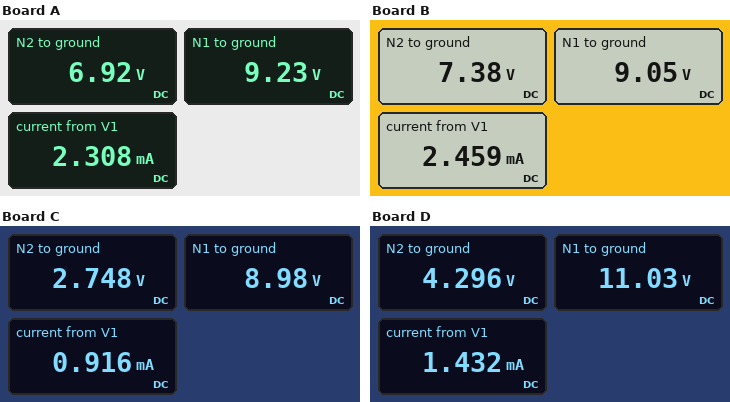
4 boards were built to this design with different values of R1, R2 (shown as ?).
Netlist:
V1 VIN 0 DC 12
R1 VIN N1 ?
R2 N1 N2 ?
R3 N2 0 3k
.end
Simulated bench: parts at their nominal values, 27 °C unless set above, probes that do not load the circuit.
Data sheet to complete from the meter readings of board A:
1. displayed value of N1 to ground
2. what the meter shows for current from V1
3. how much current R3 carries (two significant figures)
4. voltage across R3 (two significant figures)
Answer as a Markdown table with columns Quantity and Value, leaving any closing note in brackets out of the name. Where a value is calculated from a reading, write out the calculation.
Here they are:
| Quantity | Value |
|---|---|
| displayed value of N1 to ground | 9.23 V |
| what the meter shows for current from V1 | 2.308 mA |
| how much current R3 carries | (6.92 V) / 3 kΩ = 2.3 mA |
| voltage across R3 | 6.92 V = 6.9 V |
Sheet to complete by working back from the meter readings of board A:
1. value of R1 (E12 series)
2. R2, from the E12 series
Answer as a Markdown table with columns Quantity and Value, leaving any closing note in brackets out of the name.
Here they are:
| Quantity | Value |
|---|---|
| value of R1 | 1.2 kΩ |
| R2, from the E12 series | 1 kΩ |
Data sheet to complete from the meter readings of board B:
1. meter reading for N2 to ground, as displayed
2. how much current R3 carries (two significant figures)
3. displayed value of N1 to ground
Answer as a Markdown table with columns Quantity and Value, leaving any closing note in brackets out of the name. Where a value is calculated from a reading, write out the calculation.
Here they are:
| Quantity | Value |
|---|---|
| meter reading for N2 to ground, as displayed | 7.38 V |
| how much current R3 carries | (7.38 V) / 3 kΩ = 2.5 mA |
| displayed value of N1 to ground | 9.05 V |
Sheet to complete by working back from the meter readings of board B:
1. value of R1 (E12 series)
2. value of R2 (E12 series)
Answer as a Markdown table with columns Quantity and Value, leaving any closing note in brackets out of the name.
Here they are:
| Quantity | Value |
|---|---|
| value of R1 | 1.2 kΩ |
| value of R2 | 680 Ω |
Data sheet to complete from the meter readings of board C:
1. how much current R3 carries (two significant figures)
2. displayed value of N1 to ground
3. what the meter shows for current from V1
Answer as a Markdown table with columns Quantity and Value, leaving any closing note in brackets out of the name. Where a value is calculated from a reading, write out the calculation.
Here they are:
| Quantity | Value |
|---|---|
| how much current R3 carries | (2.748 V) / 3 kΩ = 920 µA |
| displayed value of N1 to ground | 8.98 V |
| what the meter shows for current from V1 | 0.916 mA |
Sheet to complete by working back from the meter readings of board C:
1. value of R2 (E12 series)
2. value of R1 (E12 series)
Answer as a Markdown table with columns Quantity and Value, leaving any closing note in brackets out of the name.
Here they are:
| Quantity | Value |
|---|---|
| value of R2 | 6.8 kΩ |
| value of R1 | 3.3 kΩ |
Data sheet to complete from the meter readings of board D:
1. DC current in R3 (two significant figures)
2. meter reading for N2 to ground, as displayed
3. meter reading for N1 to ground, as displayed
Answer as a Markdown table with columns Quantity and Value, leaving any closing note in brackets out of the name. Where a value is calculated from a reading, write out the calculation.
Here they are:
| Quantity | Value |
|---|---|
| DC current in R3 | (4.296 V) / 3 kΩ = 1.4 mA |
| meter reading for N2 to ground, as displayed | 4.296 V |
| meter reading for N1 to ground, as displayed | 11.03 V |
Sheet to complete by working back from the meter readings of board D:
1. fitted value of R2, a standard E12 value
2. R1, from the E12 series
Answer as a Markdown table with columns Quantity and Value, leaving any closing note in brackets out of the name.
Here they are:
| Quantity | Value |
|---|---|
| fitted value of R2, a standard E12 value | 4.7 kΩ |
| R1, from the E12 series | 680 Ω |
